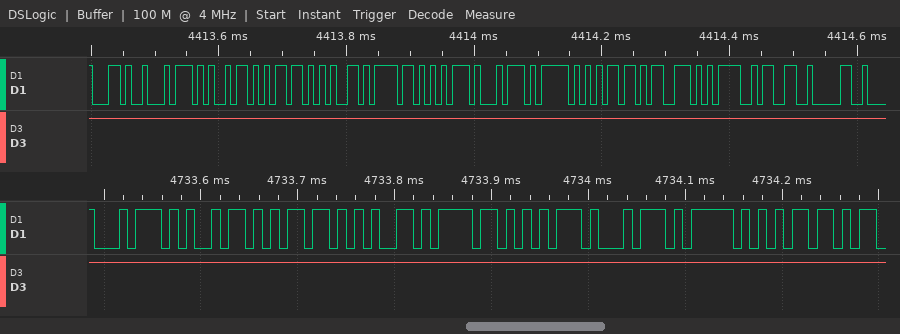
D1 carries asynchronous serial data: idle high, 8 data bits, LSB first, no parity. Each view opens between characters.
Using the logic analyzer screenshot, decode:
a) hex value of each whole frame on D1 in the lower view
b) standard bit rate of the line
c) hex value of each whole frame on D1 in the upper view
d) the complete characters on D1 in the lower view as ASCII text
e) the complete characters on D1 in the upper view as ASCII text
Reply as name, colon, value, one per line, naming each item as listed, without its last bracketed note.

hex value of each whole frame on D1 in the lower view: 74, 69, 6D, 65, 6F, 75, 74, 5F, 6D
standard bit rate of the line: 115200 baud
hex value of each whole frame on D1 in the upper view: 2C, 74, 69, 6D, 65, 6F, 75, 74, 5F, 6D, 73, 3D, 33, 30
the complete characters on D1 in the lower view as ASCII text: "timeout_m"
the complete characters on D1 in the upper view as ASCII text: ",timeout_ms=30"
